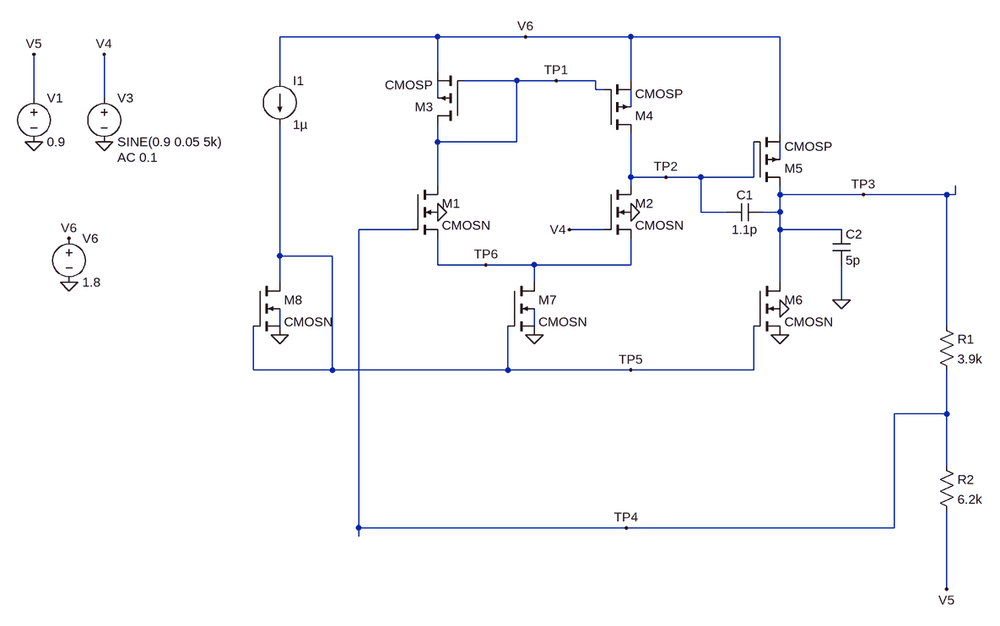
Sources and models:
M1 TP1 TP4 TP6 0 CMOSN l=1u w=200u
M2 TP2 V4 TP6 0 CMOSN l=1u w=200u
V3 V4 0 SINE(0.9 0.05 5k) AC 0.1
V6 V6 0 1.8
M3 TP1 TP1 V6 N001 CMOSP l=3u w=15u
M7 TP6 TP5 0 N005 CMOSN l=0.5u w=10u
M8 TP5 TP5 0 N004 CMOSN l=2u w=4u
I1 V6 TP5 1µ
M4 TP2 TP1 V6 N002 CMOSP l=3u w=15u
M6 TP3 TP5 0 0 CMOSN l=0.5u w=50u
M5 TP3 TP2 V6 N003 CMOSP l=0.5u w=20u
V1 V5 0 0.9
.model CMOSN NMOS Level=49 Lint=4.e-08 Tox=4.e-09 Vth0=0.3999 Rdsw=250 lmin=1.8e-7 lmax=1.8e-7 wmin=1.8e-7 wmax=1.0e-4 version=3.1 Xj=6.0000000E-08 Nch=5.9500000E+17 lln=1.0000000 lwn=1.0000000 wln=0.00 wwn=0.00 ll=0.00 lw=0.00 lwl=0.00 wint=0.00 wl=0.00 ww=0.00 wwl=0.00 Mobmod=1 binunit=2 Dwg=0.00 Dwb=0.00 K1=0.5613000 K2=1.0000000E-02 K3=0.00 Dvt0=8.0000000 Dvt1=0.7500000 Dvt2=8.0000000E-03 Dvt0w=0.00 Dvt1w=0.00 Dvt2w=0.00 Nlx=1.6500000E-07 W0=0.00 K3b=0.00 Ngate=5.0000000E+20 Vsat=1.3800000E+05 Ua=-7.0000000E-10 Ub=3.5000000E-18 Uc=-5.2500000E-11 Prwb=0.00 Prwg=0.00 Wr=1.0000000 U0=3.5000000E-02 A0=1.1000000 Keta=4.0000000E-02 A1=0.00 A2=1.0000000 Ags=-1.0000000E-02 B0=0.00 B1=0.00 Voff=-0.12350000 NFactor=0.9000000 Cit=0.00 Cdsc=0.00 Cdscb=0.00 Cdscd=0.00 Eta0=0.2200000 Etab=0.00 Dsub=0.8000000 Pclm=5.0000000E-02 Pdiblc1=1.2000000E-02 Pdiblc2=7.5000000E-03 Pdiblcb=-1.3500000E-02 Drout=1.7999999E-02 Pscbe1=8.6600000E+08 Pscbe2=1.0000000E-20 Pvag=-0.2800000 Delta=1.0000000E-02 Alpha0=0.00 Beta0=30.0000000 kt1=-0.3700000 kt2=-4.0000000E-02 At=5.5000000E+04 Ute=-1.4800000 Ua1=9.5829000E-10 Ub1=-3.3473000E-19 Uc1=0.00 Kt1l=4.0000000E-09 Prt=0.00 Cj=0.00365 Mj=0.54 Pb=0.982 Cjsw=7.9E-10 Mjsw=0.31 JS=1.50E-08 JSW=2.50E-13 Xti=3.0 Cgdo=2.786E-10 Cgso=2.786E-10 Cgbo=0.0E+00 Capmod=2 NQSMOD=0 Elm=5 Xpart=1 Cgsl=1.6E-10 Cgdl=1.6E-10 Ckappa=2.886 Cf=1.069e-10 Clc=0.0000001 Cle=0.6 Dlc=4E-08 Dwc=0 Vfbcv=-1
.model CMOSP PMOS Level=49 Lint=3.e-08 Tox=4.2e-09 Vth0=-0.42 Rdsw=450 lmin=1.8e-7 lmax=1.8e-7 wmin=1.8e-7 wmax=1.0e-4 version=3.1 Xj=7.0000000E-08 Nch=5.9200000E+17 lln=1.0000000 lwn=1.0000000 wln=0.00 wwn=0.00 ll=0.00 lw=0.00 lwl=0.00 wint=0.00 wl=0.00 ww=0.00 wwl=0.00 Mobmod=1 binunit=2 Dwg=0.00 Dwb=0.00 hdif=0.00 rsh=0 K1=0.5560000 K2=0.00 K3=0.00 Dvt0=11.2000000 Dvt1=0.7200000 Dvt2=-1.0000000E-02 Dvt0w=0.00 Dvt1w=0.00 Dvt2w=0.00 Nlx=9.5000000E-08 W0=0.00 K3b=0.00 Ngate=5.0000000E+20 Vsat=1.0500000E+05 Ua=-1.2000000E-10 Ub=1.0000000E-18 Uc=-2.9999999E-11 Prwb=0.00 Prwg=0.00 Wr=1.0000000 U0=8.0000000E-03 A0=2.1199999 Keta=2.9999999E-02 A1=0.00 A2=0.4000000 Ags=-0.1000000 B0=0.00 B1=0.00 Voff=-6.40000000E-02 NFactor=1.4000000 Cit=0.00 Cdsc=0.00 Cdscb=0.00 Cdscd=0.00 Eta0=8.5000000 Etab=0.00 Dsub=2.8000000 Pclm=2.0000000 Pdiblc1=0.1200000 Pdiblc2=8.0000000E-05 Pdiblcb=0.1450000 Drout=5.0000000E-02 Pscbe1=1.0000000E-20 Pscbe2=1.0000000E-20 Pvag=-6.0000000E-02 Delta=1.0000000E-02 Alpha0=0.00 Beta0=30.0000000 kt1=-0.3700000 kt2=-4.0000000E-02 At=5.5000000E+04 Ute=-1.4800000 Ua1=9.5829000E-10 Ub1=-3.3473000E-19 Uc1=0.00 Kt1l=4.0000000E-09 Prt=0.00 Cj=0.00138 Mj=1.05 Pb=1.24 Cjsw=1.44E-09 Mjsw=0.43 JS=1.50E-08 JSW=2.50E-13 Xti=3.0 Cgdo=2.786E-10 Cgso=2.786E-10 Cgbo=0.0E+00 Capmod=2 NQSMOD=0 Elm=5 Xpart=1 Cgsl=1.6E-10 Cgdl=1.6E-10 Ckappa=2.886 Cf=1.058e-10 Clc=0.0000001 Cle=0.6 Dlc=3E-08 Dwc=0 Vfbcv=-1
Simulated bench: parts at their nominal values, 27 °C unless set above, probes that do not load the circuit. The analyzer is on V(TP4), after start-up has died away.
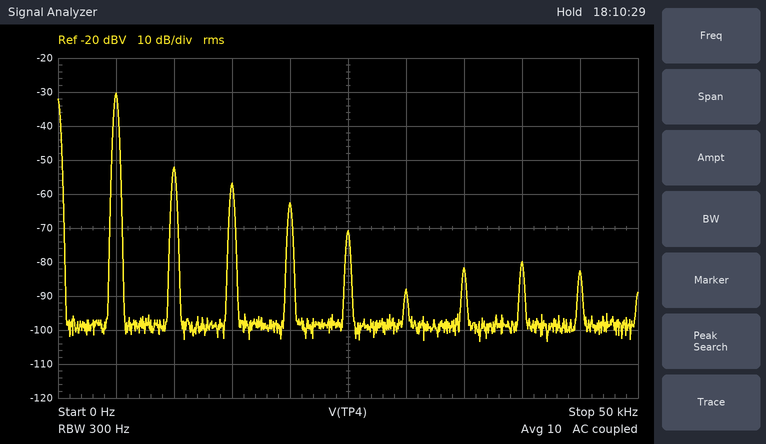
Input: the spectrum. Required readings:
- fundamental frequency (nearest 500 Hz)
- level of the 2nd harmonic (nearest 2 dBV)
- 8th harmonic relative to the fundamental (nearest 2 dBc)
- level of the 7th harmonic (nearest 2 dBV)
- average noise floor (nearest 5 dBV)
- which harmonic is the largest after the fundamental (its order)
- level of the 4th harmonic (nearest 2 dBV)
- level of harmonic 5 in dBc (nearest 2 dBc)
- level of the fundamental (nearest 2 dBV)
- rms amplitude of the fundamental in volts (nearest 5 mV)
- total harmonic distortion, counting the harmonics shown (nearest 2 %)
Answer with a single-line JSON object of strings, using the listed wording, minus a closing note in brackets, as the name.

{"fundamental frequency": "5.0 kHz", "level of the 2nd harmonic": "-52 dBV", "8th harmonic relative to the fundamental": "-50 dBc", "level of the 7th harmonic": "-82 dBV", "average noise floor": "-100 dBV", "which harmonic is the largest after the fundamental": "2", "level of the 4th harmonic": "-62 dBV", "level of harmonic 5 in dBc": "-40 dBc", "level of the fundamental": "-30 dBV", "rms amplitude of the fundamental in volts": "30 mV", "total harmonic distortion, counting the harmonics shown": "10 %"}
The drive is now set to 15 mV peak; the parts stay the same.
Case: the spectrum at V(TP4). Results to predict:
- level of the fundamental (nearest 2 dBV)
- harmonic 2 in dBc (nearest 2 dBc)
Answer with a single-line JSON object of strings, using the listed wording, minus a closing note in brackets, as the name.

{"level of the fundamental": "-40 dBV", "harmonic 2 in dBc": "-46 dBc"}
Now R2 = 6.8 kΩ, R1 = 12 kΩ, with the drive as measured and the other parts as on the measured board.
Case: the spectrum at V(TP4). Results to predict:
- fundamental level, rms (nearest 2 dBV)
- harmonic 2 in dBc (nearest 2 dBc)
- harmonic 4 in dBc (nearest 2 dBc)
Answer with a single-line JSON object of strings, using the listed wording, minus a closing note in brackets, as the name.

{"fundamental level, rms": "-30 dBV", "harmonic 2 in dBc": "-24 dBc", "harmonic 4 in dBc": "-34 dBc"}
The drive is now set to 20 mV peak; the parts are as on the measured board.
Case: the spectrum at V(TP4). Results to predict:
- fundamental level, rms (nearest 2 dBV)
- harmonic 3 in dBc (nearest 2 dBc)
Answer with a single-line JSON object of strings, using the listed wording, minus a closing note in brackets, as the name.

{"fundamental level, rms": "-38 dBV", "harmonic 3 in dBc": "-58 dBc"}
